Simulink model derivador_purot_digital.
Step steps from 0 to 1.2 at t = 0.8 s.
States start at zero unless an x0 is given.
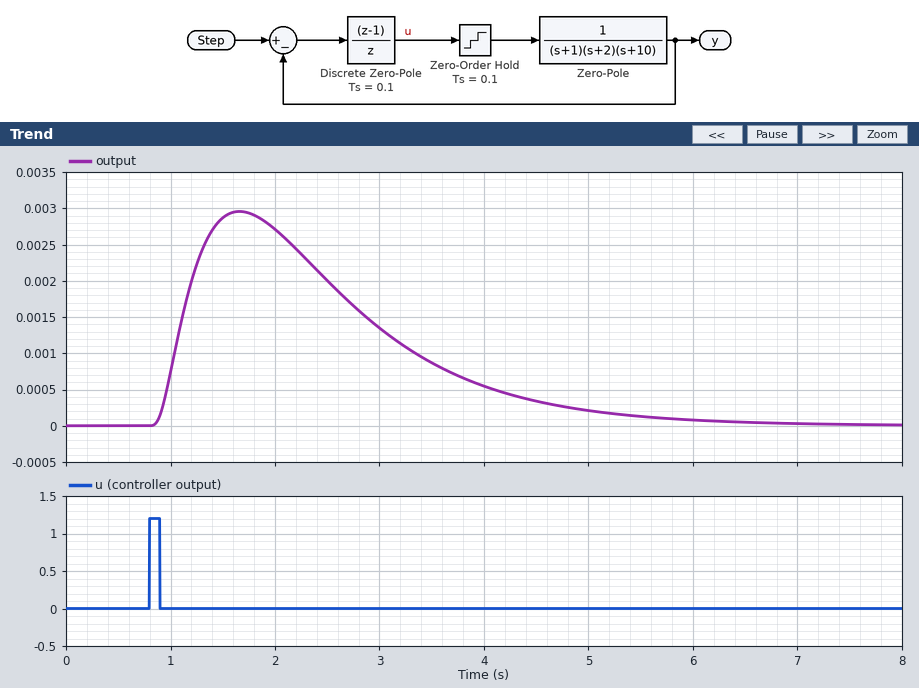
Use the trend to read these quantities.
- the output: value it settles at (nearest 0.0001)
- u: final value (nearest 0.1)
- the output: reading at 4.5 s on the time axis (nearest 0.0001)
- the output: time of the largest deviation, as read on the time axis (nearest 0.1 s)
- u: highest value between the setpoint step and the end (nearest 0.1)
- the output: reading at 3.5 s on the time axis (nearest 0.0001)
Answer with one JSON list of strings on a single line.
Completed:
["0.0000", "0.0", "0.0003", "1.7 s", "1.2", "0.0009"]
